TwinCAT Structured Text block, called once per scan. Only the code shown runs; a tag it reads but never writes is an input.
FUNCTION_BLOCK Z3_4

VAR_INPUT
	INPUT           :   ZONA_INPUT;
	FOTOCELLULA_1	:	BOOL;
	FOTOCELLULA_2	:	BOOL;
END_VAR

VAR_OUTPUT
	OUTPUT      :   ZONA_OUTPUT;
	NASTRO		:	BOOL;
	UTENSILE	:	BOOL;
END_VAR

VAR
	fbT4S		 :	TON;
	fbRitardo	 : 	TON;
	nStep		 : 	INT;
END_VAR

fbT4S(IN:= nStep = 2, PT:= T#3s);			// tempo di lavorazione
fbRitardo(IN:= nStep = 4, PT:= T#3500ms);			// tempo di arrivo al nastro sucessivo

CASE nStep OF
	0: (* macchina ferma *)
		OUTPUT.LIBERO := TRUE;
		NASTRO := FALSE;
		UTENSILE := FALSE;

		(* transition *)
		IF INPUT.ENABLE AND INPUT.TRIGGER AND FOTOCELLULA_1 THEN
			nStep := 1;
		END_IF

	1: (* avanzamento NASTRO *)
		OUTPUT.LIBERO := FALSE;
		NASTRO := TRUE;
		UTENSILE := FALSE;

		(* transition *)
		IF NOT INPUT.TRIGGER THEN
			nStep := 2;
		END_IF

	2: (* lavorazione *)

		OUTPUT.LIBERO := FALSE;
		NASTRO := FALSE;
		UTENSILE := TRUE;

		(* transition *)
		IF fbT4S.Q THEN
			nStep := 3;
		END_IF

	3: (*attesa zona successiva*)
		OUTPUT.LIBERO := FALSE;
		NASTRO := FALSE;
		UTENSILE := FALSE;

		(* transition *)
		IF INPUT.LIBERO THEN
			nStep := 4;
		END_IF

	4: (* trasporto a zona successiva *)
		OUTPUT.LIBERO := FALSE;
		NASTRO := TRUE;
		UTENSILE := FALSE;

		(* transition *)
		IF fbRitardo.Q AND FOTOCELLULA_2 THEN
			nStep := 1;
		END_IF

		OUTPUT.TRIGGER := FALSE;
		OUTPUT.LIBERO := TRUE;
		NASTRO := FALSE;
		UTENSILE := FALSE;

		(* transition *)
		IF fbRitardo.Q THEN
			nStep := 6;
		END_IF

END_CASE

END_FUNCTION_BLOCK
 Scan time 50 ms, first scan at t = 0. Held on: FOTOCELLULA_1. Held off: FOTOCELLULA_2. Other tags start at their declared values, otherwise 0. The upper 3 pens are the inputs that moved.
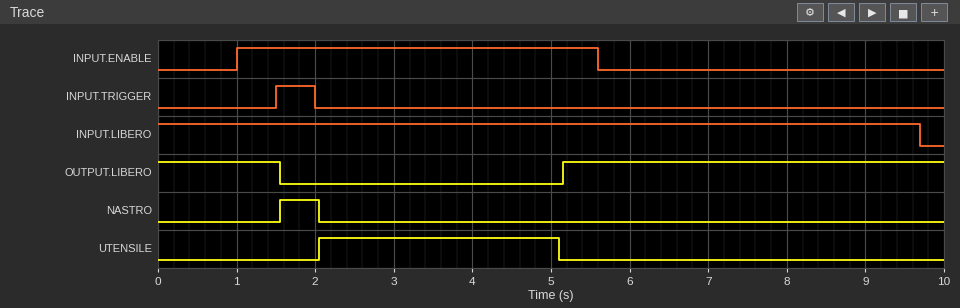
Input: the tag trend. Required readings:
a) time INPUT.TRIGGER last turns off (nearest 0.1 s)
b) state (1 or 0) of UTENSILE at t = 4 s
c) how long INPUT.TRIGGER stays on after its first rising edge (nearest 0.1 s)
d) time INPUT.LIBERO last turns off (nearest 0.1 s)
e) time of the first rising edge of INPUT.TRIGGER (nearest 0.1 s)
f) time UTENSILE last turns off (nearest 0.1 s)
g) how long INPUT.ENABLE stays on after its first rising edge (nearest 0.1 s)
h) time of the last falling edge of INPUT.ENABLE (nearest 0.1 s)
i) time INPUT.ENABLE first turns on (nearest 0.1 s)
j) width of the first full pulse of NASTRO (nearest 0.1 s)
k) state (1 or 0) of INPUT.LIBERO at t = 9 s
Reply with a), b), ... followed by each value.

a) 2.0 s
b) 1
c) 0.5 s
d) 9.7 s
e) 1.5 s
f) 5.1 s
g) 4.6 s
h) 5.6 s
i) 1.0 s
j) 0.5 s
k) 1
